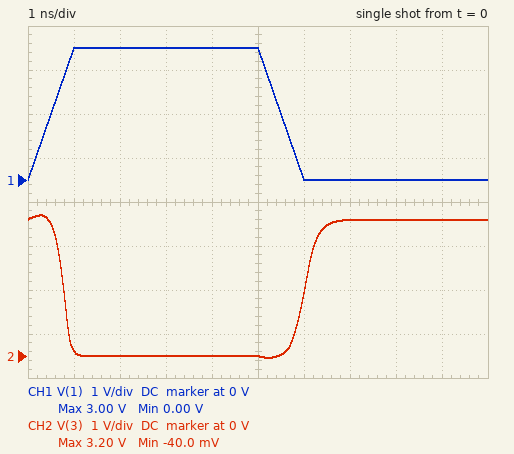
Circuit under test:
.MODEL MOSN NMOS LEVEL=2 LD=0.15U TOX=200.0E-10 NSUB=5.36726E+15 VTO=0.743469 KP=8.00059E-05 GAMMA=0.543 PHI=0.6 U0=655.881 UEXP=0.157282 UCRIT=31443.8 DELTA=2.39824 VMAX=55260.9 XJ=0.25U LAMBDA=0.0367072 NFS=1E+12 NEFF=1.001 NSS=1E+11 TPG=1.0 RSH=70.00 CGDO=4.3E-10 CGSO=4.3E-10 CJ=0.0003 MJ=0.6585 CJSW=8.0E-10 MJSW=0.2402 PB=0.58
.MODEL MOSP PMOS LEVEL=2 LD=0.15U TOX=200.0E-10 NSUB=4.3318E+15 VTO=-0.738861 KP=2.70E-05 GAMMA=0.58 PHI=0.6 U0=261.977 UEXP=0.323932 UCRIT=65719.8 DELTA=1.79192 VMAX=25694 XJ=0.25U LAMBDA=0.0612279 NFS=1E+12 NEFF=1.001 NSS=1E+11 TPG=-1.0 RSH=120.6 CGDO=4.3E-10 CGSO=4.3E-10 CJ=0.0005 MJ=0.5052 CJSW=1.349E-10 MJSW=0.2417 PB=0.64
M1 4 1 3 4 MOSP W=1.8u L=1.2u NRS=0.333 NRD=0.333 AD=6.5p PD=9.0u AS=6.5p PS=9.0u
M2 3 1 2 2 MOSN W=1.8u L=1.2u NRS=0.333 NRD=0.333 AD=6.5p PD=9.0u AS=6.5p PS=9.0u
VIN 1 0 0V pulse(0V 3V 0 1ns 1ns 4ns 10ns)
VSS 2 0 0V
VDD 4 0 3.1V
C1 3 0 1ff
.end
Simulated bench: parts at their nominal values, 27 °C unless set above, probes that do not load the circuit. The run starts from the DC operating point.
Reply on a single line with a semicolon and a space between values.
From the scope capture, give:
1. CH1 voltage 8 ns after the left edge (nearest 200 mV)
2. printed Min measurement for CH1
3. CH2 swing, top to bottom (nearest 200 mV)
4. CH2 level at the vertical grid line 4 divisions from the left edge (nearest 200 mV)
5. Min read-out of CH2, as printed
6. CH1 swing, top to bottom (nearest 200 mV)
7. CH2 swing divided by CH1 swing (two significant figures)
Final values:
0 V; 0.00 V; 3.2 V; 0 V; -40.0 mV; 3.0 V; 1.1
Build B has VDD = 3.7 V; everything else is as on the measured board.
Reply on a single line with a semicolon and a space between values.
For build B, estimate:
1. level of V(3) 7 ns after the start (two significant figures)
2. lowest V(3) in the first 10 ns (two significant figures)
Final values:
3.7 V; -19 mV
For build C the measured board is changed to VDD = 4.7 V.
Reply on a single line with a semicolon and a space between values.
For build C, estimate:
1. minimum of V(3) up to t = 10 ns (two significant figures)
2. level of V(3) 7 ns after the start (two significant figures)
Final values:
94 mV; 4.7 V
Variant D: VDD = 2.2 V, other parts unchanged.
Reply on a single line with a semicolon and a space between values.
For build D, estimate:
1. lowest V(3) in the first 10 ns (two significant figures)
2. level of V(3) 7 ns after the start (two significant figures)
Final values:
-68 mV; 2.1 V
